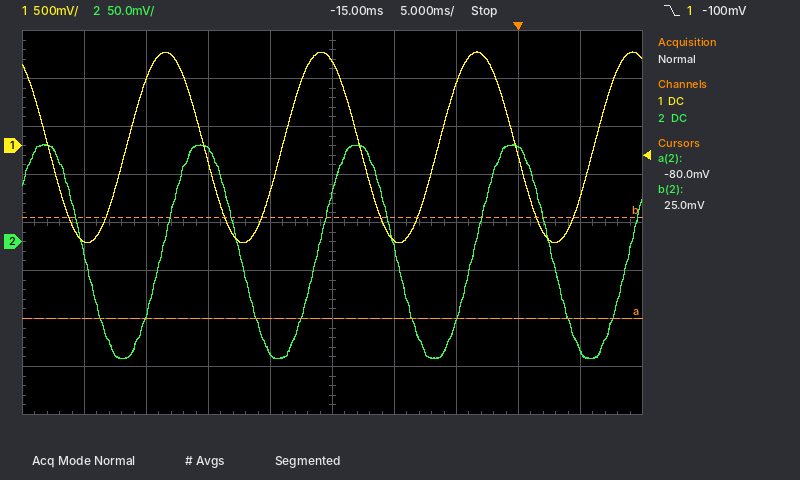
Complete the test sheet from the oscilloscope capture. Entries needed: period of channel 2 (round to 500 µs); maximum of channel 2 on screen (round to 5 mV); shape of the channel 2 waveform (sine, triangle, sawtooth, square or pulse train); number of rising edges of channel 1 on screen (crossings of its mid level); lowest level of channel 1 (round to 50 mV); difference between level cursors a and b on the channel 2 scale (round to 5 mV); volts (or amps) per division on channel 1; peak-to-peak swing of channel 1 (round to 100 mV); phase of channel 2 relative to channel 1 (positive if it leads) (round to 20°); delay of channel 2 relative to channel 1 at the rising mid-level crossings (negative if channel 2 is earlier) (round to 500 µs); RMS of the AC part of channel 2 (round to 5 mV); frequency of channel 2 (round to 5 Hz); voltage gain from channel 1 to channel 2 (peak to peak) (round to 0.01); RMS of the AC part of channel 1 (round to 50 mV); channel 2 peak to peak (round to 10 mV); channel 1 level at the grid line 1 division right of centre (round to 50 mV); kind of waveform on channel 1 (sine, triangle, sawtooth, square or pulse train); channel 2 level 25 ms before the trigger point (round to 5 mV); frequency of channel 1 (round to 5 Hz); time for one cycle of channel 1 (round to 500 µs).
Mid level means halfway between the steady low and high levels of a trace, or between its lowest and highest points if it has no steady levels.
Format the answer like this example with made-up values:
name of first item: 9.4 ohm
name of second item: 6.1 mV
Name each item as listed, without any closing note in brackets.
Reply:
period of channel 2: 12.5 ms
maximum of channel 2 on screen: 100 mV
shape of the channel 2 waveform: sine
number of rising edges of channel 1 on screen: 4
lowest level of channel 1: -1.00 V
difference between level cursors a and b on the channel 2 scale: 105 mV
volts (or amps) per division on channel 1: 500 mV
peak-to-peak swing of channel 1: 2.00 V
phase of channel 2 relative to channel 1 (positive if it leads): -80°
delay of channel 2 relative to channel 1 at the rising mid-level crossings (negative if channel 2 is earlier): +3.0 ms
RMS of the AC part of channel 2: 80 mV
frequency of channel 2: 80 Hz
voltage gain from channel 1 to channel 2 (peak to peak): 0.11
RMS of the AC part of channel 1: 700 mV
channel 2 peak to peak: 220 mV
channel 1 level at the grid line 1 division right of centre: -1.00 V
kind of waveform on channel 1: sine
channel 2 level 25 ms before the trigger point: 95 mV
frequency of channel 1: 80 Hz
time for one cycle of channel 1: 12.5 ms
